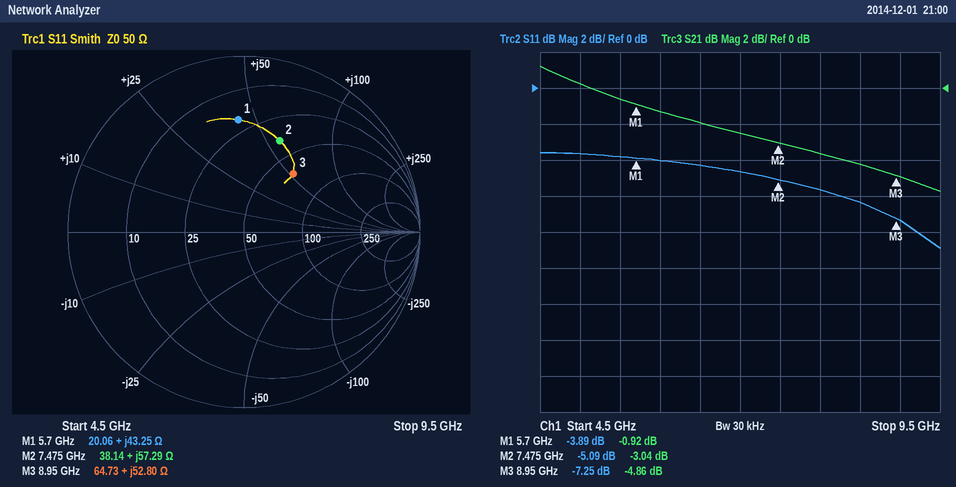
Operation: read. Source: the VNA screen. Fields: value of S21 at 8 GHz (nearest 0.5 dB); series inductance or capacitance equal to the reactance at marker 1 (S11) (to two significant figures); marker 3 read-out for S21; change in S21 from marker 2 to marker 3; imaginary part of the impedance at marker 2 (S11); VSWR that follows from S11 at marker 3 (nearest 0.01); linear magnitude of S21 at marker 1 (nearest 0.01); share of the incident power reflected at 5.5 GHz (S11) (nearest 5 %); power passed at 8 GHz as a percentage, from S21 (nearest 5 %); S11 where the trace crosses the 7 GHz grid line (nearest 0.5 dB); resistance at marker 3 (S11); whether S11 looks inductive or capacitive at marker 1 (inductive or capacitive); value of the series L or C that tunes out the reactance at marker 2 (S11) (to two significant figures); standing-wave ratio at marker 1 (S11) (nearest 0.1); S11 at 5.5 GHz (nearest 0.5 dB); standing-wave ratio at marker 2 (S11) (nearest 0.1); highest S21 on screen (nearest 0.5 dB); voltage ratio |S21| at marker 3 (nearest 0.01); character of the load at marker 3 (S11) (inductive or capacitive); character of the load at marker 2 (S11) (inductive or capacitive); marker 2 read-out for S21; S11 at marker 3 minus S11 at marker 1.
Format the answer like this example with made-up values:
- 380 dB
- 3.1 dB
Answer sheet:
- -3.5 dB
- 1.2 nH
- -4.86 dB
- -1.82 dB
- +57.29 Ω
- 2.53
- 0.90
- 40 %
- 45 %
- -4.5 dB
- 64.73 Ω
- inductive
- 370 fF
- 4.5
- -4.0 dB
- 3.5
- 1.0 dB
- 0.57
- inductive
- inductive
- -3.04 dB
- -3.36 dB
